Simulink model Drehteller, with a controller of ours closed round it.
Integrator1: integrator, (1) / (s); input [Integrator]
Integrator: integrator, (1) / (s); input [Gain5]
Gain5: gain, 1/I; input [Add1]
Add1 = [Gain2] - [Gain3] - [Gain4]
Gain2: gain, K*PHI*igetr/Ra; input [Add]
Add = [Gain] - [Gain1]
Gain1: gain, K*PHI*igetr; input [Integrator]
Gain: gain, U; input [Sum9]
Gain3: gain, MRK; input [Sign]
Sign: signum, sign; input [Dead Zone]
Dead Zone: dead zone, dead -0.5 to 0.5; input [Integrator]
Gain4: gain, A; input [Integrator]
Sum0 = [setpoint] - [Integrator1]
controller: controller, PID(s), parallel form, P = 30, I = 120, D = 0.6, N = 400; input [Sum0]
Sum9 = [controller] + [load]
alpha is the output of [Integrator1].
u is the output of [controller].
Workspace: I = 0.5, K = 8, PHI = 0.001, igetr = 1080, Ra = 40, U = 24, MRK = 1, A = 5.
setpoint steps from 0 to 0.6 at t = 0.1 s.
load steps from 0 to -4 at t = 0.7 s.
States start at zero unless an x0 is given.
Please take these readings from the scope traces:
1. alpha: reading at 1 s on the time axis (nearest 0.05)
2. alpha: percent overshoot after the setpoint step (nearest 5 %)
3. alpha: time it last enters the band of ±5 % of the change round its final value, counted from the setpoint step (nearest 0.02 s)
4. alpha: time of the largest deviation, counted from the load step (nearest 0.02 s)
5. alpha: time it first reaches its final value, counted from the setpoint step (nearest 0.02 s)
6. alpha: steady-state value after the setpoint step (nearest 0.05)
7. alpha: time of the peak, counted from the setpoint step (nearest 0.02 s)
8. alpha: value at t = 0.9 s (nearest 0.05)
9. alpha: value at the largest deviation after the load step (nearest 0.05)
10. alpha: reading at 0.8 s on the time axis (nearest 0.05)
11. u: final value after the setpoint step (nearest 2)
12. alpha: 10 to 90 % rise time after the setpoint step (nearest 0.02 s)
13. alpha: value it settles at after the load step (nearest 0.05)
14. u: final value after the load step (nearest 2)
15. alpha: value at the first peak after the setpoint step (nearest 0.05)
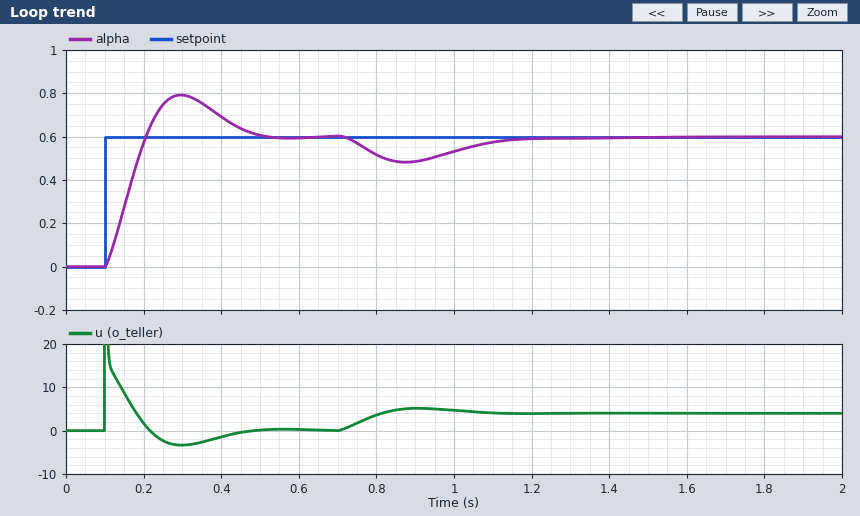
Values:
0.55
30 %
0.36 s
0.18 s
0.10 s
0.60
0.20 s
0.50
0.50
0.50
0
0.08 s
0.60
4
0.80
